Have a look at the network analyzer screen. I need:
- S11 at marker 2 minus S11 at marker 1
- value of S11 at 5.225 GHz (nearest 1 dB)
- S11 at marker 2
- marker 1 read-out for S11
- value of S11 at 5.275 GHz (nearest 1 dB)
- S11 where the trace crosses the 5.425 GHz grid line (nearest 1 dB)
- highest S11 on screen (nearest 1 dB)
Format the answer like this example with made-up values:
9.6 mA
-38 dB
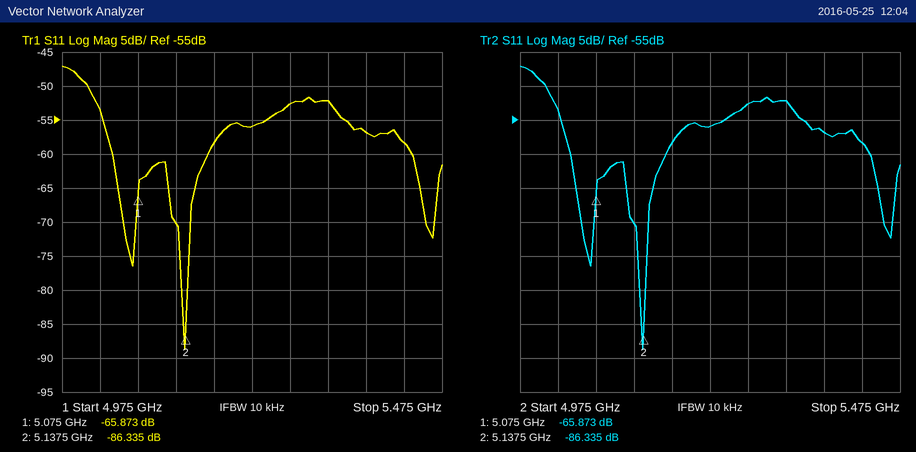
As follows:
-20.462 dB
-56 dB
-86.335 dB
-65.873 dB
-53 dB
-58 dB
-47 dB
